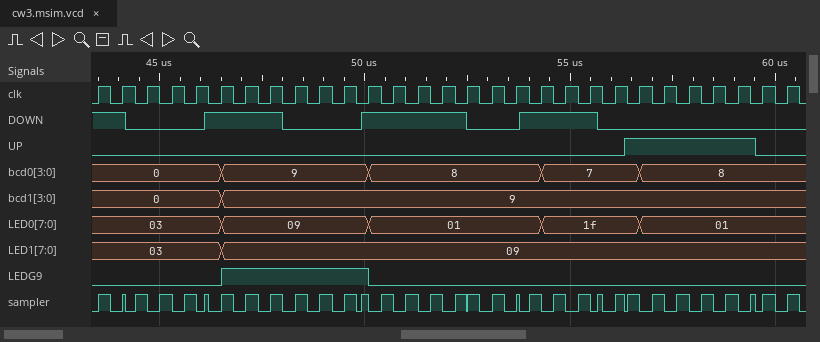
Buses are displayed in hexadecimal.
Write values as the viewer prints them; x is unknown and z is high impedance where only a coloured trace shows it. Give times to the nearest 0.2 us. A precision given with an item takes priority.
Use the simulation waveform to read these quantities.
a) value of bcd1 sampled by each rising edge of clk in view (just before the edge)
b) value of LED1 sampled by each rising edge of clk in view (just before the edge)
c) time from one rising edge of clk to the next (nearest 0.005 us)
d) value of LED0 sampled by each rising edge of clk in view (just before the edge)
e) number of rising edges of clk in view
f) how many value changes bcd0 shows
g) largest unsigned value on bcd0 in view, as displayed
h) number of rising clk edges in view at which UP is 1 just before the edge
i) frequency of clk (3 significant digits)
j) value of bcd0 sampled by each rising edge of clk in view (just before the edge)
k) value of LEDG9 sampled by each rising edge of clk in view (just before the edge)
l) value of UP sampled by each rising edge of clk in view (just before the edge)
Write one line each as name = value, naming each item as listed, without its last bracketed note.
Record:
value of bcd1 sampled by each rising edge of clk in view = 0, 0, 0, 0, 0, 0, 9, 9, 9, 9, 9, 9, 9, 9, 9, 9, 9, 9, 9, 9, 9, 9, 9, 9, 9, 9, 9, 9, 9
value of LED1 sampled by each rising edge of clk in view = 03, 03, 03, 03, 03, 03, 09, 09, 09, 09, 09, 09, 09, 09, 09, 09, 09, 09, 09, 09, 09, 09, 09, 09, 09, 09, 09, 09, 09
time from one rising edge of clk to the next = 0.6 us
value of LED0 sampled by each rising edge of clk in view = 03, 03, 03, 03, 03, 03, 09, 09, 09, 09, 09, 09, 01, 01, 01, 01, 01, 01, 01, 1f, 1f, 1f, 1f, 01, 01, 01, 01, 01, 01
number of rising edges of clk in view = 29
how many value changes bcd0 shows = 4
largest unsigned value on bcd0 in view, as displayed = 9
number of rising clk edges in view at which UP is 1 just before the edge = 5
frequency of clk = 1.67 MHz
value of bcd0 sampled by each rising edge of clk in view = 0, 0, 0, 0, 0, 0, 9, 9, 9, 9, 9, 9, 8, 8, 8, 8, 8, 8, 8, 7, 7, 7, 7, 8, 8, 8, 8, 8, 8
value of LEDG9 sampled by each rising edge of clk in view = 0 0 0 0 0 0 1 1 1 1 1 1 0 0 0 0 0 0 0 0 0 0 0 0 0 0 0 0 0
value of UP sampled by each rising edge of clk in view = 0 0 0 0 0 0 0 0 0 0 0 0 0 0 0 0 0 0 0 0 0 0 1 1 1 1 1 0 0
